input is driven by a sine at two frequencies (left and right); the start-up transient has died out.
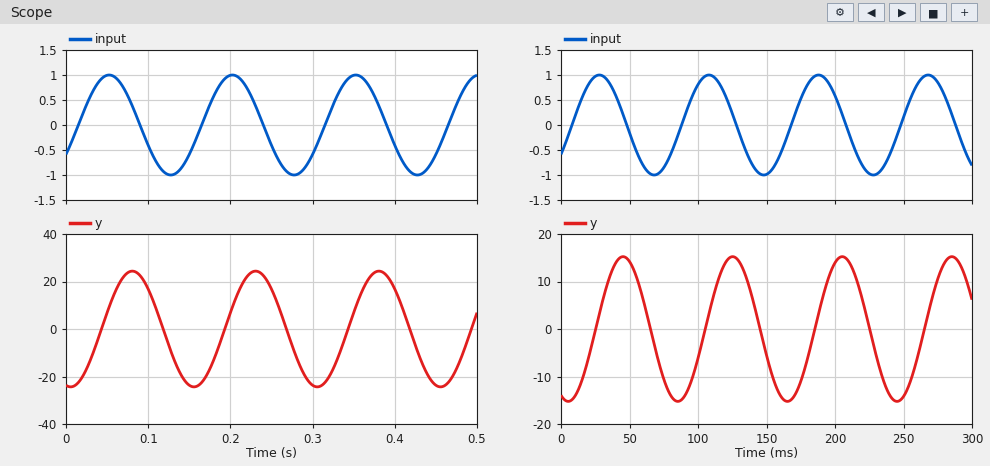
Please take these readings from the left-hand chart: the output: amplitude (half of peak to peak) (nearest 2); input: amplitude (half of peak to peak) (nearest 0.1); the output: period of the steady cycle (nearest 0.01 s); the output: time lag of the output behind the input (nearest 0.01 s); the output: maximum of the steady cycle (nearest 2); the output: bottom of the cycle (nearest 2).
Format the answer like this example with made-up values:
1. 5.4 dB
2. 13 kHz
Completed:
1. 24
2. 1.0
3. 0.15 s
4. 0.03 s
5. 24
6. -24
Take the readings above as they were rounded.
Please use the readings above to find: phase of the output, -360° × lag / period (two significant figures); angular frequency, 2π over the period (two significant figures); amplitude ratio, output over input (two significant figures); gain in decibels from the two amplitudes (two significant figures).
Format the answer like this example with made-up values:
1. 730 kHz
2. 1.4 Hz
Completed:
1. -72°
2. 42 rad/s
3. 24
4. 28 dB
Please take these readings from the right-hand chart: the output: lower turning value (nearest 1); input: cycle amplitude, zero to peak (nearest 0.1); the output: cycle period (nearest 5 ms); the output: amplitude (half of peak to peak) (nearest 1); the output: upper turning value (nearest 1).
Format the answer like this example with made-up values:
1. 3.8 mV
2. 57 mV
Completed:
1. -15
2. 1.0
3. 80 ms
4. 15
5. 15
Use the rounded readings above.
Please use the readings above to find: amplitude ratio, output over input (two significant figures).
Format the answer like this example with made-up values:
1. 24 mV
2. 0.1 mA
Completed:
1. 15
